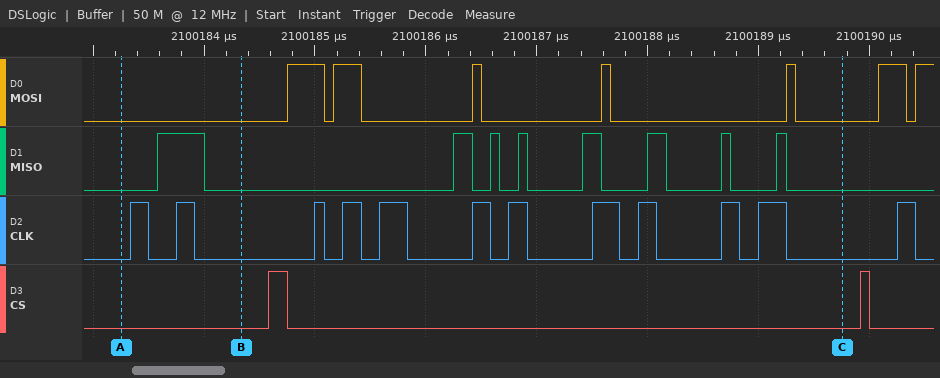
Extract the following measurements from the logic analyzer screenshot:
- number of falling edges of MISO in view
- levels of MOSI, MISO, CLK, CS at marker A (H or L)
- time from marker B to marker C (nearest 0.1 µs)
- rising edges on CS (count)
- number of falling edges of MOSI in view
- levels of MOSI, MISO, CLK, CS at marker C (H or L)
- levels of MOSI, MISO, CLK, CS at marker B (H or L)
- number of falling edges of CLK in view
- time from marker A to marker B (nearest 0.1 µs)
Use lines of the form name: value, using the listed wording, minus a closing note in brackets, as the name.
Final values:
number of falling edges of MISO in view: 8
levels of MOSI, MISO, CLK, CS at marker A: MOSI=L, MISO=L, CLK=L, CS=L
time from marker B to marker C: 5.4 µs
rising edges on CS: 2
number of falling edges of MOSI in view: 6
levels of MOSI, MISO, CLK, CS at marker C: MOSI=L, MISO=L, CLK=L, CS=L
levels of MOSI, MISO, CLK, CS at marker B: MOSI=L, MISO=L, CLK=L, CS=L
number of falling edges of CLK in view: 12
time from marker A to marker B: 1.1 µs
